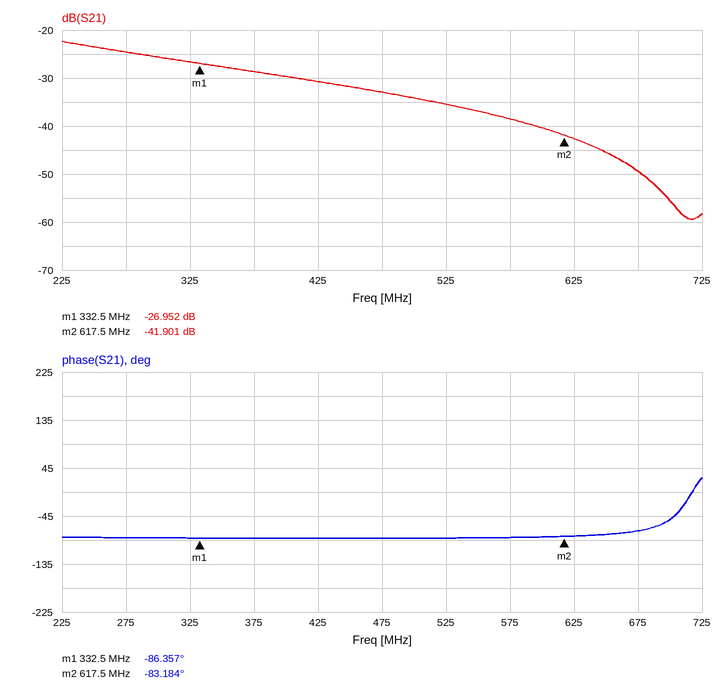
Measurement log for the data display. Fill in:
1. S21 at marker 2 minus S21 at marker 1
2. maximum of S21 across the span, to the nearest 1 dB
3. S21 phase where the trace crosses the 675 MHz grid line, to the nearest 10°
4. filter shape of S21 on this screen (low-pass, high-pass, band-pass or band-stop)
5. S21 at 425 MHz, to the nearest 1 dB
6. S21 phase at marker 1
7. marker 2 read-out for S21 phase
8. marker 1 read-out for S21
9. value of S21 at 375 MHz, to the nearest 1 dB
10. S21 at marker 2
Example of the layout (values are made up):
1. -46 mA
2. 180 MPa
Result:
1. -14.949 dB
2. -22 dB
3. -70°
4. low-pass
5. -31 dB
6. -86.357°
7. -83.184°
8. -26.952 dB
9. -29 dB
10. -41.901 dB
